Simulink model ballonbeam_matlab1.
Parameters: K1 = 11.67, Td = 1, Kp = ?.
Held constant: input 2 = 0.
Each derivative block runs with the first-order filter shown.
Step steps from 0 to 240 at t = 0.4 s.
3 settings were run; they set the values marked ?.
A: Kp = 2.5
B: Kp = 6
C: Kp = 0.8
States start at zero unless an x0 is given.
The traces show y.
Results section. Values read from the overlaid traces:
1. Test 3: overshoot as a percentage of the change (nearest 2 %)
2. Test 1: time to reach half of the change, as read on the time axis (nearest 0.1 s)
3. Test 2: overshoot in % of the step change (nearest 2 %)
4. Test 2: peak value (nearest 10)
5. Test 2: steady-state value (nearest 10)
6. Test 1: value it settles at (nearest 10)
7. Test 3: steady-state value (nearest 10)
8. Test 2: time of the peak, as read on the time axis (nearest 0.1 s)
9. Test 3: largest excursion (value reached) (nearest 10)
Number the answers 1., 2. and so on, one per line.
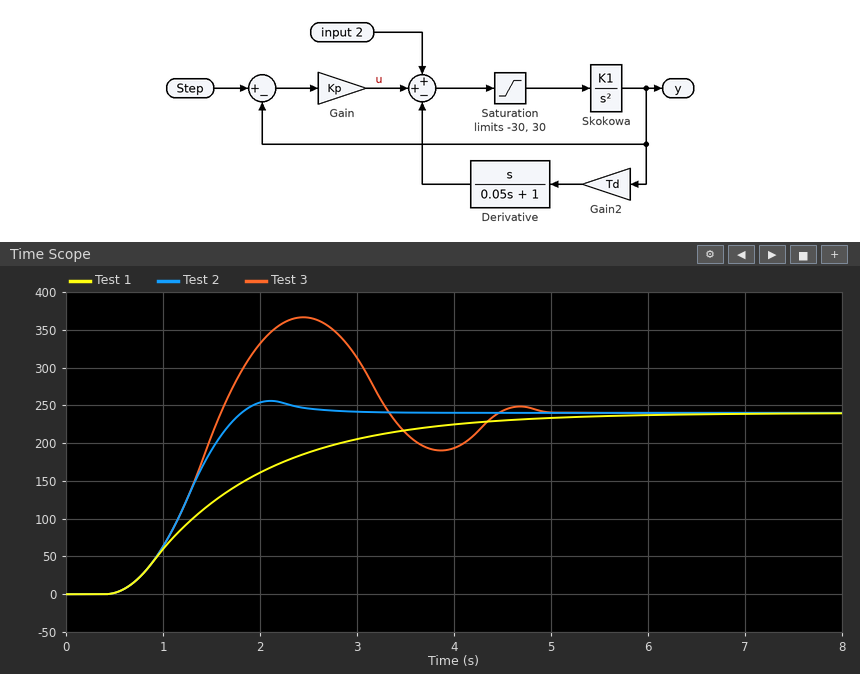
1. 52 %
2. 1.5 s
3. 6 %
4. 260
5. 240
6. 240
7. 240
8. 2.1 s
9. 370
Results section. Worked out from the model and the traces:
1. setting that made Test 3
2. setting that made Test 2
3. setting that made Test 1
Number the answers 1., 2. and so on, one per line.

1. B
2. A
3. C
